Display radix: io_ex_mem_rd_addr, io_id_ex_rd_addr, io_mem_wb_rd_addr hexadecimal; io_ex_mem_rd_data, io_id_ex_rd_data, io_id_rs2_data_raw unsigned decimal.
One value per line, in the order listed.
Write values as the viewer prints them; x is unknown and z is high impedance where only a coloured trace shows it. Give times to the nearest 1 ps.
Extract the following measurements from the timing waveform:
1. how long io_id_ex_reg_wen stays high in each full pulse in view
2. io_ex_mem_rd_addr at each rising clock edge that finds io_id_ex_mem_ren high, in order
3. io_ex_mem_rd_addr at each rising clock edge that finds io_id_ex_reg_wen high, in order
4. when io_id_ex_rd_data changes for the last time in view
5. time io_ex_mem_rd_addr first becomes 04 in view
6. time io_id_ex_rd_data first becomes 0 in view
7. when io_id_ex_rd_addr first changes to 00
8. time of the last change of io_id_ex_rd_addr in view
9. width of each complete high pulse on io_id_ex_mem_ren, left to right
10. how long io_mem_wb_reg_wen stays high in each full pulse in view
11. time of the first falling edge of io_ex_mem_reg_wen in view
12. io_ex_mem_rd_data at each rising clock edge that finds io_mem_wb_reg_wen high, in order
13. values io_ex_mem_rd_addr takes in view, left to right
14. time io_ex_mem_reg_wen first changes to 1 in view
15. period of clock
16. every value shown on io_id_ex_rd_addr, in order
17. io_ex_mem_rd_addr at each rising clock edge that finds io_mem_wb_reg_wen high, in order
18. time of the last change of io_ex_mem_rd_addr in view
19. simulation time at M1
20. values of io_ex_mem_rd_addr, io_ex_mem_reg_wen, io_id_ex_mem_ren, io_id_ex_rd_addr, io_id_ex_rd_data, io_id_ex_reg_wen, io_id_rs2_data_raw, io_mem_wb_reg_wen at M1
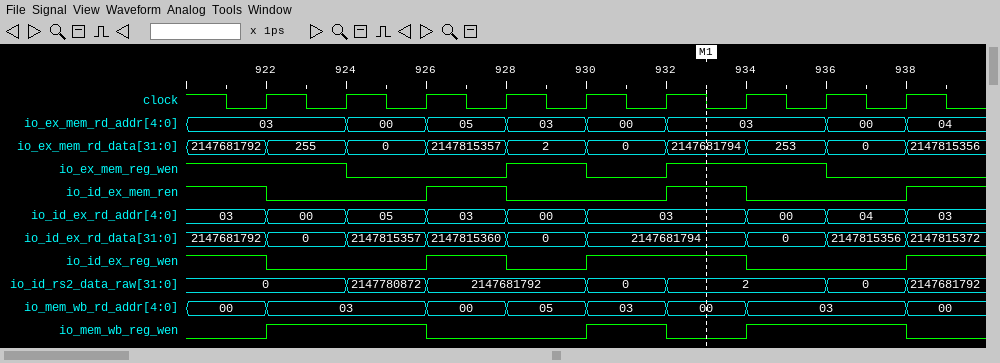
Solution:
2 ps, 4 ps
03, 05, 03
03, 05, 00, 03
938 ps
938 ps
922 ps
922 ps
938 ps
2 ps, 2 ps
4 ps, 2 ps, 4 ps
924 ps
255, 0, 0, 253, 0
03, 00, 05, 03, 00, 03, 00, 04
928 ps
2 ps
03, 00, 05, 03, 00, 03, 00, 04, 03
03, 00, 00, 03, 00
938 ps
933 ps
io_ex_mem_rd_addr=03, io_ex_mem_reg_wen=1, io_id_ex_mem_ren=1, io_id_ex_rd_addr=03, io_id_ex_rd_data=2147681794, io_id_ex_reg_wen=1, io_id_rs2_data_raw=2, io_mem_wb_reg_wen=0
